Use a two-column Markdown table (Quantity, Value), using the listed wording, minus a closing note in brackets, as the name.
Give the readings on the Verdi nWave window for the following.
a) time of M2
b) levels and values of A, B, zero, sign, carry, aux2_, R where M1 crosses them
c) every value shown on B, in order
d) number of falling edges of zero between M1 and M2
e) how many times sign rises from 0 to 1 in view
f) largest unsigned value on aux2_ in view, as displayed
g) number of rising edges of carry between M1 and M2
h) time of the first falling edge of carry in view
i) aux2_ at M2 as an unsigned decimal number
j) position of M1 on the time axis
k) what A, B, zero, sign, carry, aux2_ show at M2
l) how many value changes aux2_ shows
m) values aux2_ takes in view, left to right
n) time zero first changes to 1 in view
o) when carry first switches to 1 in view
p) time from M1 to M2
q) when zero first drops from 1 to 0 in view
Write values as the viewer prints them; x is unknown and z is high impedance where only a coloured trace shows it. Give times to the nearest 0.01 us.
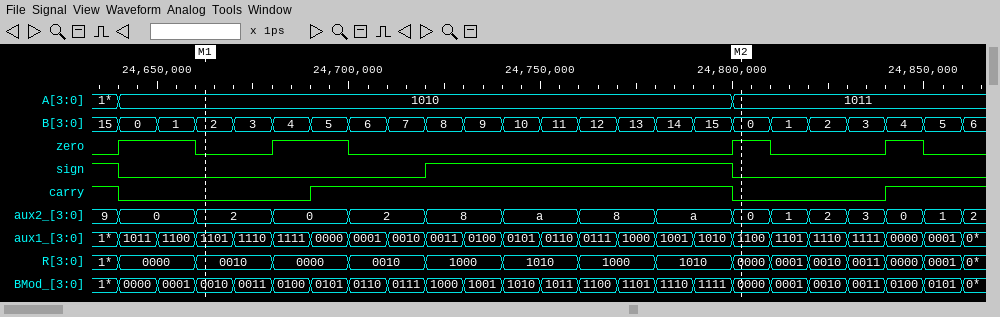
| Quantity | Value |
|---|---|
| time of M2 | 24.8 us |
| levels and values of A, B, zero, sign, carry, aux2_, R where M1 crosses them | A=1010, B=2, zero=0, sign=0, carry=0, aux2_=2, R=0010 |
| every value shown on B, in order | 15, 0, 1, 2, 3, 4, 5, 6, 7, 8, 9, 10, 11, 12, 13, 14, 15, 0, 1, 2, 3, 4, 5, 6 |
| number of falling edges of zero between M1 and M2 | 1 |
| how many times sign rises from 0 to 1 in view | 1 |
| largest unsigned value on aux2_ in view, as displayed | a |
| number of rising edges of carry between M1 and M2 | 1 |
| time of the first falling edge of carry in view | 24.64 us |
| aux2_ at M2 as an unsigned decimal number | 0 |
| position of M1 on the time axis | 24.66 us |
| what A, B, zero, sign, carry, aux2_ show at M2 | A=1011, B=0, zero=1, sign=0, carry=0, aux2_=0 |
| how many value changes aux2_ shows | 15 |
| values aux2_ takes in view, left to right | 9, 0, 2, 0, 2, 8, a, 8, a, 0, 1, 2, 3, 0, 1, 2 |
| time zero first changes to 1 in view | 24.64 us |
| when carry first switches to 1 in view | 24.69 us |
| time from M1 to M2 | 0.14 us |
| when zero first drops from 1 to 0 in view | 24.66 us |
